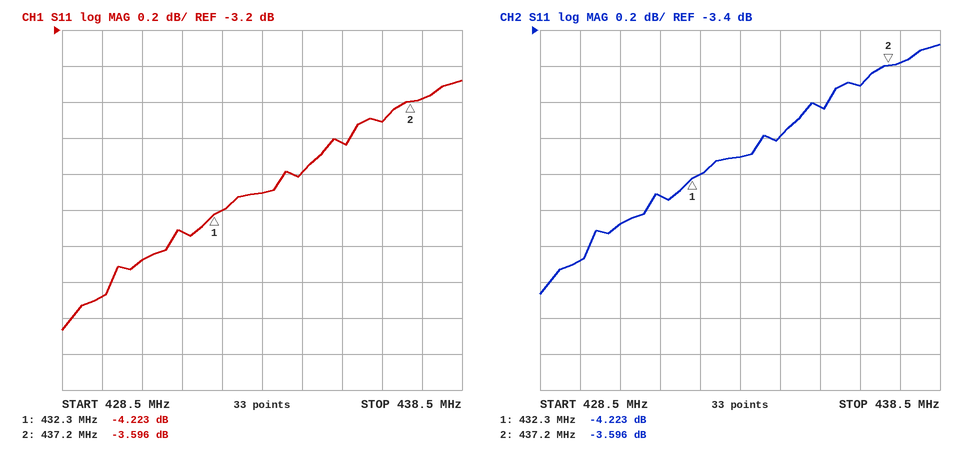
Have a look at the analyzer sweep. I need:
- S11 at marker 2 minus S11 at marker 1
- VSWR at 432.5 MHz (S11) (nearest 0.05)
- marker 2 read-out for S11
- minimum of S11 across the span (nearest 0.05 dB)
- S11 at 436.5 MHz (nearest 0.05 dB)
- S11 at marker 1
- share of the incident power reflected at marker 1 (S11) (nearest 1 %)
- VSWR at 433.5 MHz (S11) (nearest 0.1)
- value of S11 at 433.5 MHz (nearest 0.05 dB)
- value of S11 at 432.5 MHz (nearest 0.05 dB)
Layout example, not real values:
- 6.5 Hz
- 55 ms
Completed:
- 0.627 dB
- 4.20
- -3.596 dB
- -4.85 dB
- -3.70 dB
- -4.223 dB
- 38 %
- 4.3
- -4.10 dB
- -4.20 dB
